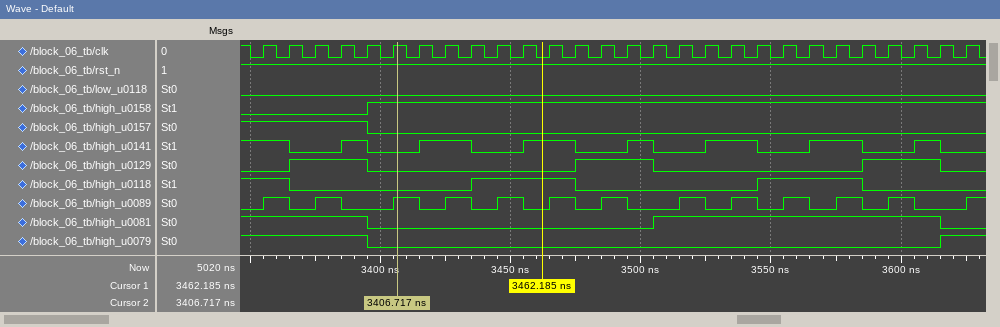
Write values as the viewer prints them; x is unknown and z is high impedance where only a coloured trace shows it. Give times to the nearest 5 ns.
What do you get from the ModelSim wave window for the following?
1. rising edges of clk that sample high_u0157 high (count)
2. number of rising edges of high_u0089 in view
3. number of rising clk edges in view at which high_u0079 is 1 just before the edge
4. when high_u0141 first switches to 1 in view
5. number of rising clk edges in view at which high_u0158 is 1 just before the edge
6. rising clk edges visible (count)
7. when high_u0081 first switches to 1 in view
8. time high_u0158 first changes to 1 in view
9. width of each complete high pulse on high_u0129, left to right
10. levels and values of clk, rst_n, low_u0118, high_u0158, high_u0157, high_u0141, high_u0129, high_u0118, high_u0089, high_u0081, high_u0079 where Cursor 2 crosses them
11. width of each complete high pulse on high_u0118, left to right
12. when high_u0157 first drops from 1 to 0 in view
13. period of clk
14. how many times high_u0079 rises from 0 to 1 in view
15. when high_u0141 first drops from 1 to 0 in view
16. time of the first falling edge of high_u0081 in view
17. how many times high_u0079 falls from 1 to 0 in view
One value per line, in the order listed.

5
13
6
3385 ns
23
28
3505 ns
3395 ns
30 ns, 30 ns, 30 ns
clk=1, rst_n=1, low_u0118=0, high_u0158=1, high_u0157=0, high_u0141=0, high_u0129=0, high_u0118=0, high_u0089=1, high_u0081=0, high_u0079=0
40 ns, 40 ns
3395 ns
10 ns
1
3365 ns
3395 ns
1
